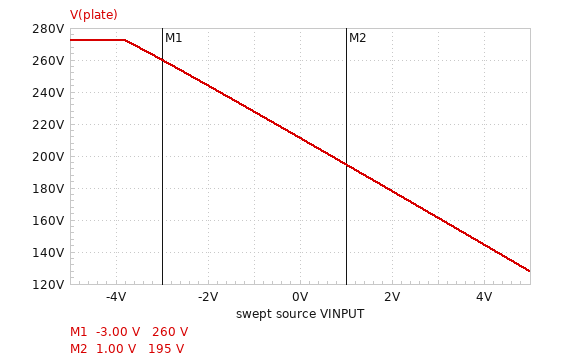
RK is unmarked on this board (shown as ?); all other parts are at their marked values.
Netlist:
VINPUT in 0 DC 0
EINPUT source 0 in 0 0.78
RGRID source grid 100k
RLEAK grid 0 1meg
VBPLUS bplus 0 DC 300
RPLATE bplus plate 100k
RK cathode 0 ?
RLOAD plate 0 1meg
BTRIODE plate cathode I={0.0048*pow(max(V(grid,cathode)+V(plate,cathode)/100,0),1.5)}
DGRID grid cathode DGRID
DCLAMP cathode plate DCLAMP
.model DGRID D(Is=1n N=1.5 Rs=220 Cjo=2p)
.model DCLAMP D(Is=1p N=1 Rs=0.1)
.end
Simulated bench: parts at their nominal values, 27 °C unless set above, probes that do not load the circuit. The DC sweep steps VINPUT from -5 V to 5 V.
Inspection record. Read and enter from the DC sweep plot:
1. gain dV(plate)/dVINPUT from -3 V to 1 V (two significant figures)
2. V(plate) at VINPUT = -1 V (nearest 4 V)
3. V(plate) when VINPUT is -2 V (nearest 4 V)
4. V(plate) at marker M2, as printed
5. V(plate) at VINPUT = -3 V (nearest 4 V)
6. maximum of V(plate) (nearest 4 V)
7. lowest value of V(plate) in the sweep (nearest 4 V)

-16 V/V
228 V
244 V
195 V
260 V
272 V
128 V
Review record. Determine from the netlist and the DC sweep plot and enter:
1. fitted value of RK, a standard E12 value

2.7 kΩ
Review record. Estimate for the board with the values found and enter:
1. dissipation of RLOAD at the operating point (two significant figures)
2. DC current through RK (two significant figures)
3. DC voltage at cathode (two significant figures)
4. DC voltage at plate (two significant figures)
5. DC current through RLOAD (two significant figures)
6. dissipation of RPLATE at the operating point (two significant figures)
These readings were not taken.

45 mW
680 µA
1.8 V
210 V
210 µA
79 mW
